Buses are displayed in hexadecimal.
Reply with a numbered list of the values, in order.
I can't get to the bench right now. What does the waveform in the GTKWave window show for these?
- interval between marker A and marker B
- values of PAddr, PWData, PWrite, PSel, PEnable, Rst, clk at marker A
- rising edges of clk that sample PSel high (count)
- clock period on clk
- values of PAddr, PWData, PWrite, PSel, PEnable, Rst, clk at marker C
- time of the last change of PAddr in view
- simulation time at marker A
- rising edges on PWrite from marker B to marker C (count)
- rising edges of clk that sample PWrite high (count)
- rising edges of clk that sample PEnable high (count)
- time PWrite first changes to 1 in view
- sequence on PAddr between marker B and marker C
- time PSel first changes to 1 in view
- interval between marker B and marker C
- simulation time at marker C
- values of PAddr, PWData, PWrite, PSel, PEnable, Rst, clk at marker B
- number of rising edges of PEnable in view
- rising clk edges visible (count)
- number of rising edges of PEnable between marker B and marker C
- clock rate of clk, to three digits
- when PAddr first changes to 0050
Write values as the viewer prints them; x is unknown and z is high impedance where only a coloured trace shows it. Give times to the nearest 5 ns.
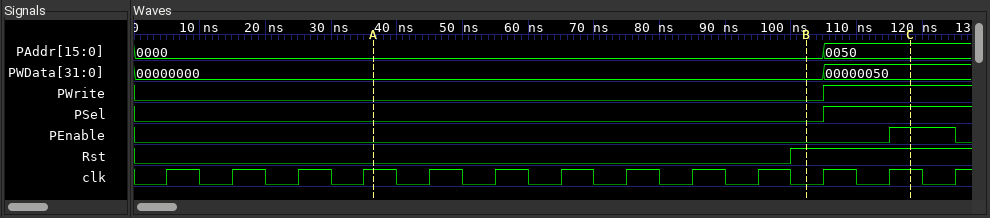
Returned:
1. 65 ns
2. PAddr=0000, PWData=00000000, PWrite=0, PSel=0, PEnable=0, Rst=0, clk=1
3. 2
4. 10 ns
5. PAddr=0050, PWData=00000050, PWrite=1, PSel=1, PEnable=1, Rst=1, clk=1
6. 105 ns
7. 35 ns
8. 1
9. 2
10. 1
11. 105 ns
12. 0000, 0050
13. 105 ns
14. 15 ns
15. 120 ns
16. PAddr=0000, PWData=00000000, PWrite=0, PSel=0, PEnable=0, Rst=1, clk=0
17. 1
18. 13
19. 1
20. 100 MHz
21. 105 ns
